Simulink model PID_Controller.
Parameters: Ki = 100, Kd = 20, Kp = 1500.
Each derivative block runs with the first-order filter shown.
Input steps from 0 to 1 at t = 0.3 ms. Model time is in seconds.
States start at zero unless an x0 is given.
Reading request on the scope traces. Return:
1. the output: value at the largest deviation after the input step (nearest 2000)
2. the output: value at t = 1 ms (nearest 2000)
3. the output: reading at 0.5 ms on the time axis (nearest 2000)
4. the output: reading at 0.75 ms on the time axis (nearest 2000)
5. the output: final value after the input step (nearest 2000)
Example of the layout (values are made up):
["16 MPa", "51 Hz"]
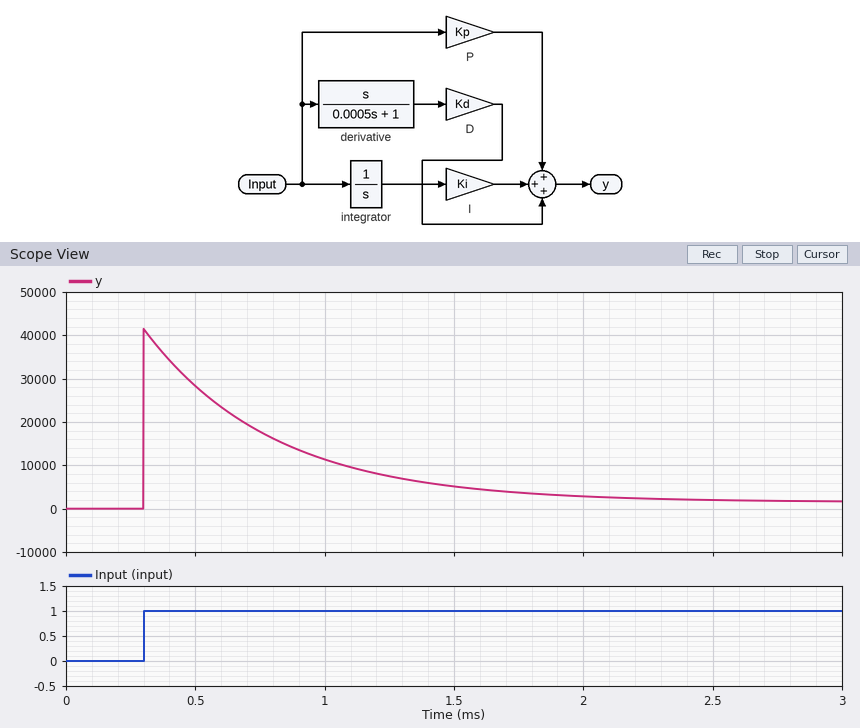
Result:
["42000", "12000", "28000", "18000", "2000"]
